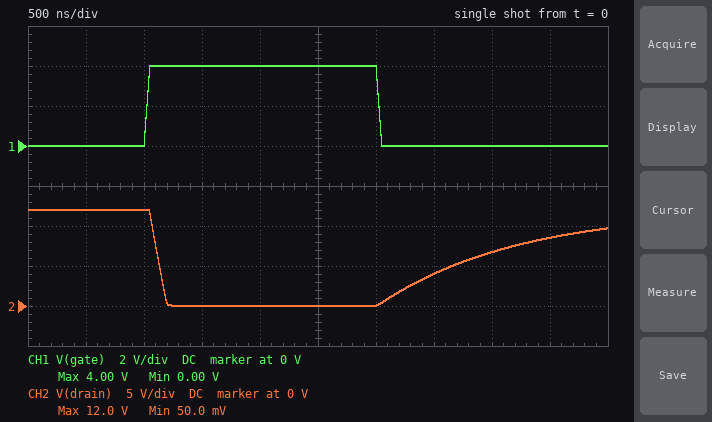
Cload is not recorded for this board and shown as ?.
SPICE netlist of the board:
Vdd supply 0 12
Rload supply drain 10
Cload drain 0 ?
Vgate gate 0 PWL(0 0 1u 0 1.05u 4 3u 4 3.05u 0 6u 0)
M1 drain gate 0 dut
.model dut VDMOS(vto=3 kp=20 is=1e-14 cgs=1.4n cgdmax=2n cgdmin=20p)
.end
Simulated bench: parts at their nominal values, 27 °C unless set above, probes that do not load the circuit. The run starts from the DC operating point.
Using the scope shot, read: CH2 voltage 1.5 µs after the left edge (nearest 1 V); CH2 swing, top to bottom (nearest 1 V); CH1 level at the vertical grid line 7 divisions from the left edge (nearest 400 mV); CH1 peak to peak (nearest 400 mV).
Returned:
0 V
12 V
0 V
4.0 V
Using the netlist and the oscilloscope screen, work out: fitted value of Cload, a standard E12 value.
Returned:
120 nF
